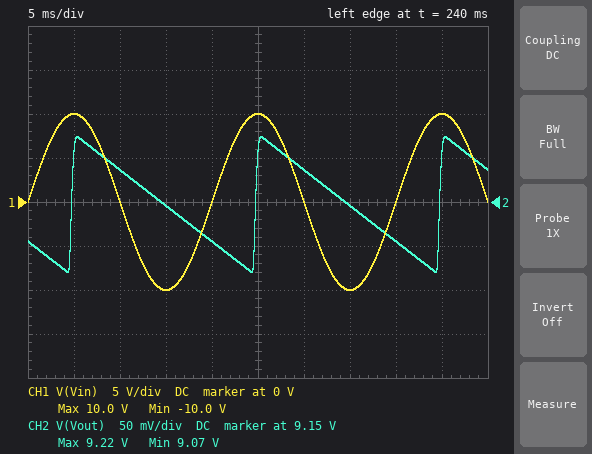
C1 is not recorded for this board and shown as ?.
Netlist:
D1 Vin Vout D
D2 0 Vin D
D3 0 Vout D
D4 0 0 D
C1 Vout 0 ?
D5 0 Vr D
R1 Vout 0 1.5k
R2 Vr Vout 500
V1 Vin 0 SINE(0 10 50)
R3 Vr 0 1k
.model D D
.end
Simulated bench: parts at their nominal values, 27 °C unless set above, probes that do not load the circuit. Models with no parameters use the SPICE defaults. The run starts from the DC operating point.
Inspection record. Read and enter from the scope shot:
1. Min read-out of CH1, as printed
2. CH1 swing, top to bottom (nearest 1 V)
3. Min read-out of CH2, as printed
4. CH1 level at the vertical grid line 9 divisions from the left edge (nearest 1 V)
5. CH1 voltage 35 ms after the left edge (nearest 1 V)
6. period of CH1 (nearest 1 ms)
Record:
-10.0 V
20 V
9.07 V
10 V
-10 V
20 ms
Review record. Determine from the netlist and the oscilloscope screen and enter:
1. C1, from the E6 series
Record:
1.5 mF
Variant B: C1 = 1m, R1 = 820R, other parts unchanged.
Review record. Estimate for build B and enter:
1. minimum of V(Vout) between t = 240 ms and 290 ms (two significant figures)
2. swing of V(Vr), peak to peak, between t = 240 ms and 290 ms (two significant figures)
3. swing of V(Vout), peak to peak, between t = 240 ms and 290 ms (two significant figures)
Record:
8.9 V
210 mV
320 mV
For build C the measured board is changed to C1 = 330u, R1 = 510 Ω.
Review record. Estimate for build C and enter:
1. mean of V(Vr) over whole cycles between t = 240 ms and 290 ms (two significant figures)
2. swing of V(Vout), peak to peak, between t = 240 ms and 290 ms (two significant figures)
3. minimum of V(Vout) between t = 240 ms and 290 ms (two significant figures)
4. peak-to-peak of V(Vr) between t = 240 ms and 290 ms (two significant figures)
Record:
5.8 V
1.2 V
8.0 V
830 mV
